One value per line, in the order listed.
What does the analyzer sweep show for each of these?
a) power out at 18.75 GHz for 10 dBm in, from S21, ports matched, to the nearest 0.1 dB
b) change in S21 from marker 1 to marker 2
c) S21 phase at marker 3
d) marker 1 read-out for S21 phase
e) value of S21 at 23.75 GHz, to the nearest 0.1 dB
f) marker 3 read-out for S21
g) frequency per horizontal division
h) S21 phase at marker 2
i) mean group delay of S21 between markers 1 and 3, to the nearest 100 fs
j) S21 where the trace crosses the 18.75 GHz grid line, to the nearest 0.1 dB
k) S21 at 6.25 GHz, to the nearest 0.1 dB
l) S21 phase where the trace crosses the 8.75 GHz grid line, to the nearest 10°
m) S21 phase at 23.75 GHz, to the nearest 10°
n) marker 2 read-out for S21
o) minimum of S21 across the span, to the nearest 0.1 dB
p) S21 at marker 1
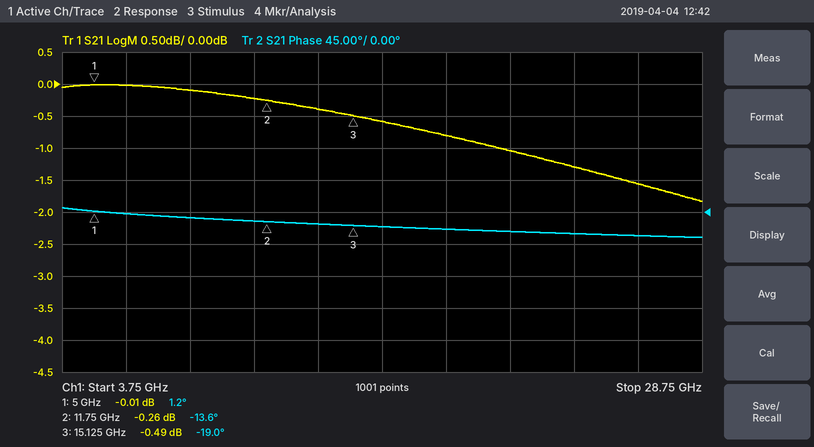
9.2 dBm
-0.25 dB
-19.0°
1.2°
-1.3 dB
-0.49 dB
2.5 GHz
-13.6°
5.5 ps
-0.8 dB
0.0 dB
-10°
-30°
-0.26 dB
-1.8 dB
-0.01 dB
